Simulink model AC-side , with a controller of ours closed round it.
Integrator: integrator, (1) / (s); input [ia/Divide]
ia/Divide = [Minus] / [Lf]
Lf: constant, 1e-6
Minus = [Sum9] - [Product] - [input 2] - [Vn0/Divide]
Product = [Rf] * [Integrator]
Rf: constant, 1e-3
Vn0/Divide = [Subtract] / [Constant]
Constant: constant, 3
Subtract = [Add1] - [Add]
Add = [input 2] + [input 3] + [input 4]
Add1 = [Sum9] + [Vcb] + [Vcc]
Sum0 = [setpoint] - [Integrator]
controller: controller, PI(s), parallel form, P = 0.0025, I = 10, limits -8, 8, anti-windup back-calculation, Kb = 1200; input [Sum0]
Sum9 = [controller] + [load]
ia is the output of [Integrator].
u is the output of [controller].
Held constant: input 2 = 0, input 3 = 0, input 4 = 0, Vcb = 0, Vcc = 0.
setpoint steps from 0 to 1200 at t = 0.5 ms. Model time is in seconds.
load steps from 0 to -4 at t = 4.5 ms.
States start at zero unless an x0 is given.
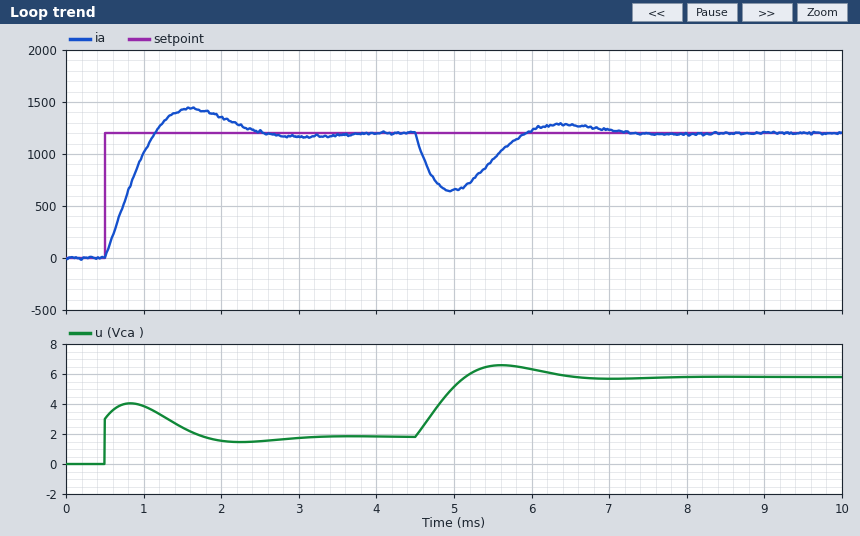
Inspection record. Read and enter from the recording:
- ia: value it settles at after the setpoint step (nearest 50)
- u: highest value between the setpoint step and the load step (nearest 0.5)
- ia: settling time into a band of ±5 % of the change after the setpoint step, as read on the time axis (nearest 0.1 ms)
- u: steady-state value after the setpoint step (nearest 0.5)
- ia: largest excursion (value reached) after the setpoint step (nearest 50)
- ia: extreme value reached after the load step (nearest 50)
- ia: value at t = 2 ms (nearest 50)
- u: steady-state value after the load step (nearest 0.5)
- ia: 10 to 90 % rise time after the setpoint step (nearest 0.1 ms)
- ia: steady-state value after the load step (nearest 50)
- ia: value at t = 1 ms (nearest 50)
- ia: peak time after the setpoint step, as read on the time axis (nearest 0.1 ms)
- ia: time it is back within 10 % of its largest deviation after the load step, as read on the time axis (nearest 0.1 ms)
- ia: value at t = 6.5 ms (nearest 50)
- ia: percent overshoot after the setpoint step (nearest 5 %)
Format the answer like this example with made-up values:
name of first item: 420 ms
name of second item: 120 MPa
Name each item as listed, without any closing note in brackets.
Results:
ia: value it settles at after the setpoint step: 1200
u: highest value between the setpoint step and the load step: 4.0
ia: settling time into a band of ±5 % of the change after the setpoint step, as read on the time axis: 2.3 ms
u: steady-state value after the setpoint step: 2.0
ia: largest excursion (value reached) after the setpoint step: 1450
ia: extreme value reached after the load step: 650
ia: value at t = 2 ms: 1350
u: steady-state value after the load step: 6.0
ia: 10 to 90 % rise time after the setpoint step: 0.5 ms
ia: steady-state value after the load step: 1200
ia: value at t = 1 ms: 1000
ia: peak time after the setpoint step, as read on the time axis: 1.6 ms
ia: time it is back within 10 % of its largest deviation after the load step, as read on the time axis: 6.8 ms
ia: value at t = 6.5 ms: 1300
ia: percent overshoot after the setpoint step: 20 %
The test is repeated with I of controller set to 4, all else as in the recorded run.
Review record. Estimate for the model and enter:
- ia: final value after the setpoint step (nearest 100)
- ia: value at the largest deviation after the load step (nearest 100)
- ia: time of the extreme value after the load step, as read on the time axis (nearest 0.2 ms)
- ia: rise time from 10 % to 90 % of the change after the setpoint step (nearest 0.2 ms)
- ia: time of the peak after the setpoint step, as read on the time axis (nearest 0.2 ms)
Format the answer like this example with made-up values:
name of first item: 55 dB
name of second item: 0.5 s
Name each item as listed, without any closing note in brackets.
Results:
ia: final value after the setpoint step: 1200
ia: value at the largest deviation after the load step: 500
ia: time of the extreme value after the load step, as read on the time axis: 5.2 ms
ia: rise time from 10 % to 90 % of the change after the setpoint step: 0.8 ms
ia: time of the peak after the setpoint step, as read on the time axis: 2.4 ms
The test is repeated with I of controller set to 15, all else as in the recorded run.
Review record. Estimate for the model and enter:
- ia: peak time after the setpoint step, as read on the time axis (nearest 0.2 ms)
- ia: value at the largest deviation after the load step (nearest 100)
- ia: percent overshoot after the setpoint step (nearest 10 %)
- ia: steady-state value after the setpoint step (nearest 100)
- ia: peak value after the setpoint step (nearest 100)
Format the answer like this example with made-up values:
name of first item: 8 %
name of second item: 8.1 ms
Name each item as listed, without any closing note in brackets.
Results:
ia: peak time after the setpoint step, as read on the time axis: 1.4 ms
ia: value at the largest deviation after the load step: 700
ia: percent overshoot after the setpoint step: 30 %
ia: steady-state value after the setpoint step: 1200
ia: peak value after the setpoint step: 1500
